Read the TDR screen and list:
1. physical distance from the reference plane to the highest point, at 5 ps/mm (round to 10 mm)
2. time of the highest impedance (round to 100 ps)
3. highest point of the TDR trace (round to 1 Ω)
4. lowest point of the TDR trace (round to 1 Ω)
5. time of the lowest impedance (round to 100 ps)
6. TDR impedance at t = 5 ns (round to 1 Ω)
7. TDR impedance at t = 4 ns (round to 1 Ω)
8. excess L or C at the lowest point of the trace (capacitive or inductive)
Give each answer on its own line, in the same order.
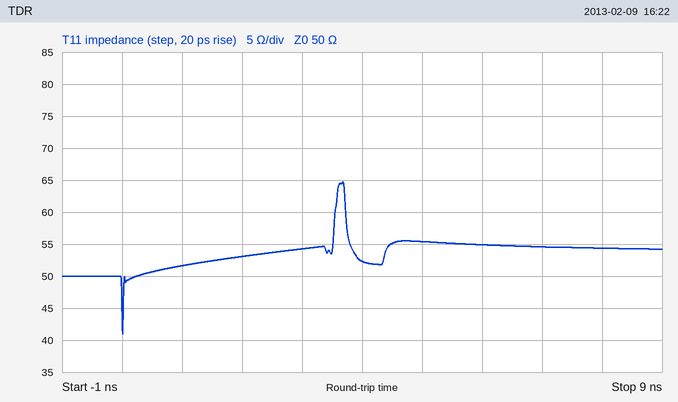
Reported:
370 mm
3.7 ns
65 Ω
41 Ω
0.0 ns
55 Ω
52 Ω
capacitive
